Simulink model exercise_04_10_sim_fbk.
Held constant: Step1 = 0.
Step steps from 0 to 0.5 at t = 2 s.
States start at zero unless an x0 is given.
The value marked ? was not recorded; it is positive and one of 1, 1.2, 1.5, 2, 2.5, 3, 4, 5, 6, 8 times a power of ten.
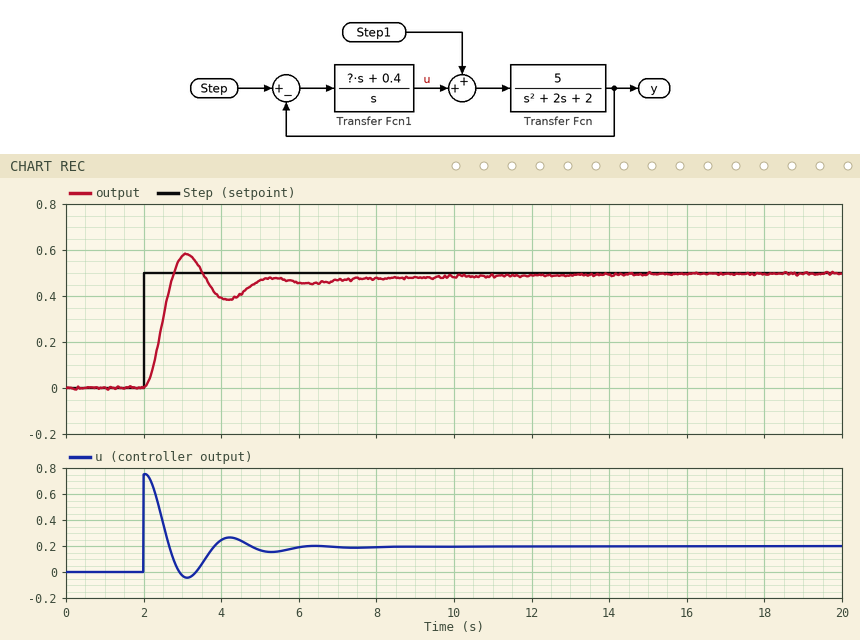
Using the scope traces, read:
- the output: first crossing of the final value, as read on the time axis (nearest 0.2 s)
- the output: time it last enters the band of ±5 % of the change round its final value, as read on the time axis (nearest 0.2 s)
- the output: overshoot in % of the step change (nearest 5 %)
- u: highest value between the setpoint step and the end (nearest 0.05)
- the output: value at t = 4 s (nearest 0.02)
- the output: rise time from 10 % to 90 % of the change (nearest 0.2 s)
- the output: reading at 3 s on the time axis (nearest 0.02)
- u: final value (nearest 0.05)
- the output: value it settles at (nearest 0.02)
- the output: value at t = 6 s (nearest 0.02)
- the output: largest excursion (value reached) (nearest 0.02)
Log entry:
2.8 s
7.4 s
15 %
0.75
0.40
0.6 s
0.58
0.20
0.50
0.46
0.58
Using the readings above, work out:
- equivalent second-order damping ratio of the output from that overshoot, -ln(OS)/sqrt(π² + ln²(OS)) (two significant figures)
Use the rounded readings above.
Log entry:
0.52
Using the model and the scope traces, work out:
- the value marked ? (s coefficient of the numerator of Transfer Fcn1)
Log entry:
1.5
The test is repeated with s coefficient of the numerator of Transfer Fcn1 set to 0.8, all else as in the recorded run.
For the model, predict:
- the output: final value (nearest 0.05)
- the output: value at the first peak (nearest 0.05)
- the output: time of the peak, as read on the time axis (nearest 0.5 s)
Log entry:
0.50
0.55
3.5 s
